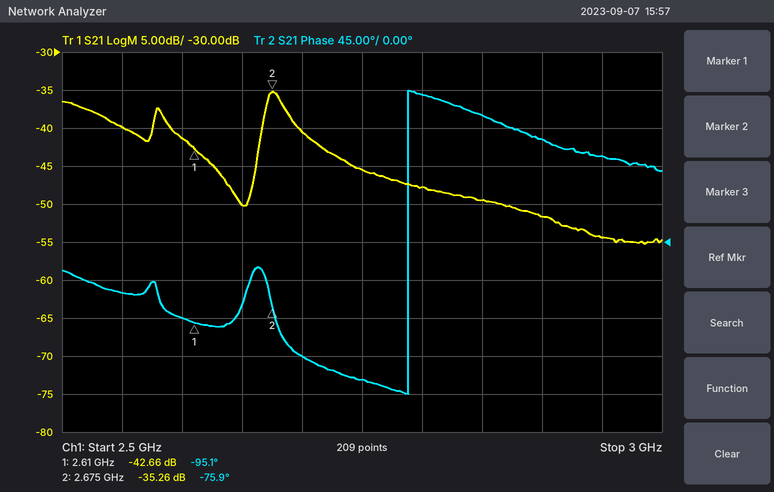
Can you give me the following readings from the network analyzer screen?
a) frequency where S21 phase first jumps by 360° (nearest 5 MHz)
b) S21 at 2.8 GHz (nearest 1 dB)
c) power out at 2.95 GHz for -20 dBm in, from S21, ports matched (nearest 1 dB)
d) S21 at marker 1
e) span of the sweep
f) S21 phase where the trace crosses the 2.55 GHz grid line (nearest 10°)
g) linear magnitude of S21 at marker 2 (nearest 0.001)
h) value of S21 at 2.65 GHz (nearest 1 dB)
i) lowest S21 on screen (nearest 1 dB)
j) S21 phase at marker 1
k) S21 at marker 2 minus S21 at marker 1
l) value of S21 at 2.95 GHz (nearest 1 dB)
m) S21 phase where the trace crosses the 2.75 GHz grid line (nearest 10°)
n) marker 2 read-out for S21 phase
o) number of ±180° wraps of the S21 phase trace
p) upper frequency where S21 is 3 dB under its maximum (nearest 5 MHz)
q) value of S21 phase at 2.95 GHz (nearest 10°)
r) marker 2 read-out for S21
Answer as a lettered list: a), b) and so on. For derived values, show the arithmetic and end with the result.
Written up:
a) 2.790 GHz
b) -48 dB
c) -20 dBm + (-54 dB) = -74 dBm
d) -42.66 dB
e) 500 MHz
f) -60°
g) 10^(-35.26/20) ≈ 0.017
h) -50 dB
i) -55 dB
j) -95.1°
k) -35.26 − (-42.66) = 7.40 dB
l) -54 dB
m) -160°
n) -75.9°
o) 1
p) 2.690 GHz
q) 100°
r) -35.26 dB
